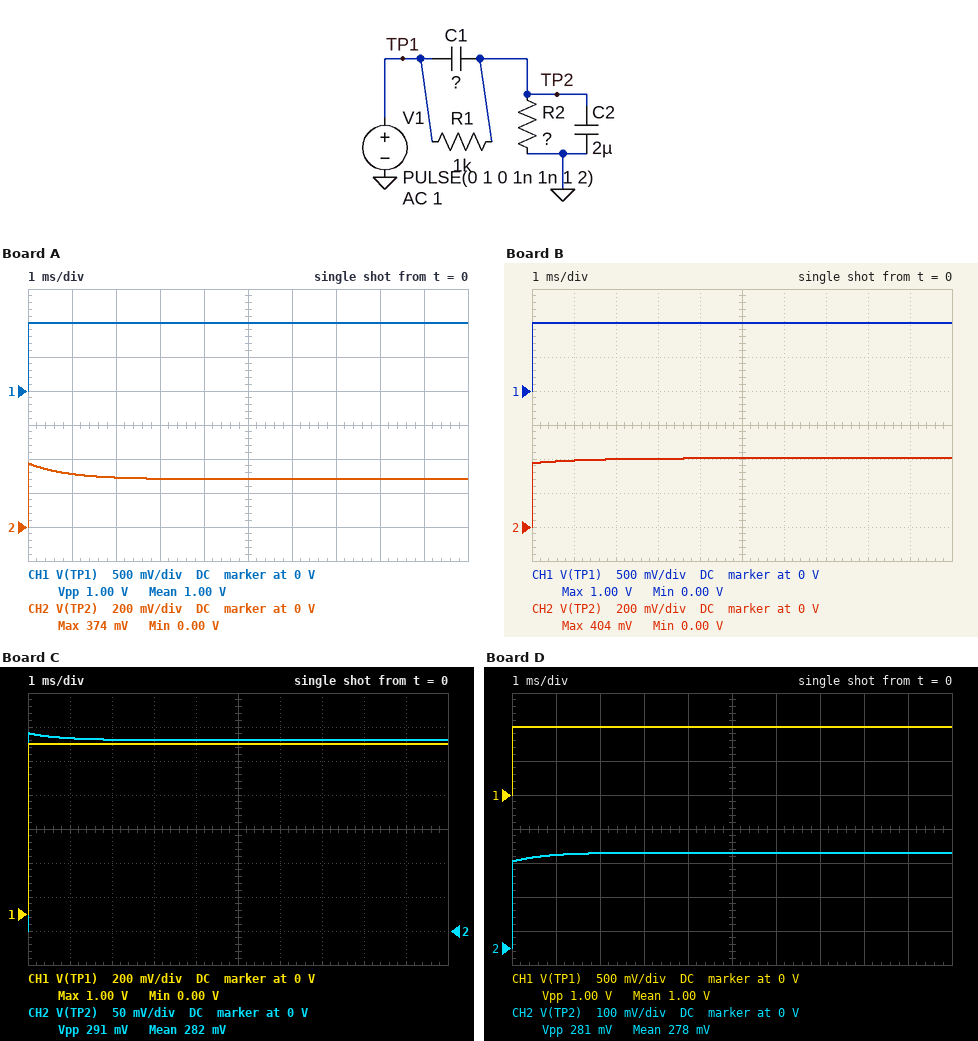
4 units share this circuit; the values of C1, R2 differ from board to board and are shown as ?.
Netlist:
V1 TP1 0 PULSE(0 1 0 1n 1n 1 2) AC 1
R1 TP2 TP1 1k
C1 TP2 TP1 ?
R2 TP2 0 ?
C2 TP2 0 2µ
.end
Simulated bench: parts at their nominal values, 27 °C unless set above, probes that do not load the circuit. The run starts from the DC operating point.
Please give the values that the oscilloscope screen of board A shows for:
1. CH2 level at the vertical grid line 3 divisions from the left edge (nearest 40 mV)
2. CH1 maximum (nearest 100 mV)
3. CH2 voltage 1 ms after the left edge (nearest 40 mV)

280 mV
1.0 V
320 mV
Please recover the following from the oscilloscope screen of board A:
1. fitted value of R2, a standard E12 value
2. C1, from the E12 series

390 Ω
1.2 µF
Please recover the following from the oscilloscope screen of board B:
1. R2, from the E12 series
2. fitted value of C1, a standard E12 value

680 Ω
1.2 µF
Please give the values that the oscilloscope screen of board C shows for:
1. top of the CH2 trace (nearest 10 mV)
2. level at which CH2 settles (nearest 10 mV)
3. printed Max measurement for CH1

290 mV
280 mV
1.00 V
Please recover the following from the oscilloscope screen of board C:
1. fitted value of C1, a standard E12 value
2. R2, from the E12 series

820 nF
390 Ω
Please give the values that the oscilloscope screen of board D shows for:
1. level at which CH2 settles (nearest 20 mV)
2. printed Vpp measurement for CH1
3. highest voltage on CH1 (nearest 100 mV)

280 mV
1.00 V
1.0 V
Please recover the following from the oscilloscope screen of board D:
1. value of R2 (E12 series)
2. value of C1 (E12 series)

390 Ω
680 nF
